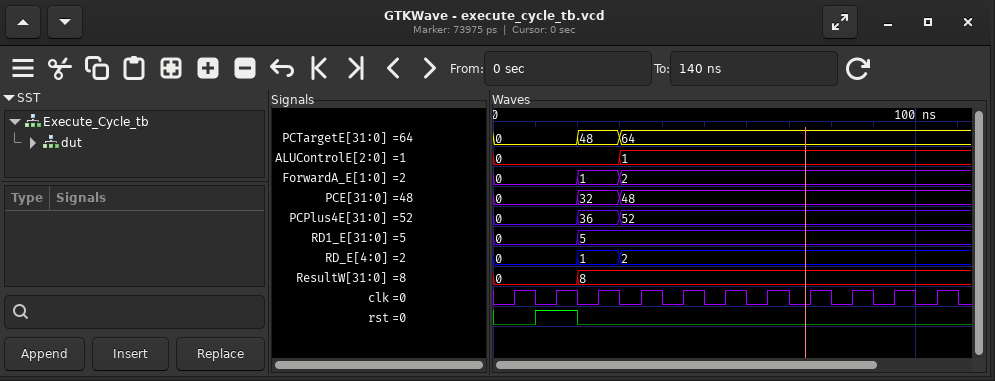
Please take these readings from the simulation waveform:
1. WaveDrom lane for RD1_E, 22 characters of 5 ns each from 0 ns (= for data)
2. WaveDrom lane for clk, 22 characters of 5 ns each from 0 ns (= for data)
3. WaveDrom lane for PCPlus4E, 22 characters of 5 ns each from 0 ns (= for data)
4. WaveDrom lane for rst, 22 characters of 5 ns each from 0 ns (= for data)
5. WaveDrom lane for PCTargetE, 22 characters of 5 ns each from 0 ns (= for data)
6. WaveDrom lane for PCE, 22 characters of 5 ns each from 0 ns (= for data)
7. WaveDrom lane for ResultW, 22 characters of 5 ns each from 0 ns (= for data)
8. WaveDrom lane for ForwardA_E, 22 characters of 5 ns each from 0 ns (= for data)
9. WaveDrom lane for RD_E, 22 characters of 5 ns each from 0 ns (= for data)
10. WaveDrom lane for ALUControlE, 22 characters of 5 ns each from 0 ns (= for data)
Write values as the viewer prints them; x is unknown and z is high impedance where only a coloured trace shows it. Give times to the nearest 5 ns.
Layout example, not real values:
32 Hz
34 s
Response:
{name: 'RD1_E', wave: '=...=.................', data: '0 5'}
{name: 'clk', wave: '0101010101010101010101'}
{name: 'PCPlus4E', wave: '=...=.=...............', data: '0 36 52'}
{name: 'rst', wave: '0.1.0.................'}
{name: 'PCTargetE', wave: '=...=.=...............', data: '0 48 64'}
{name: 'PCE', wave: '=...=.=...............', data: '0 32 48'}
{name: 'ResultW', wave: '=...=.................', data: '0 8'}
{name: 'ForwardA_E', wave: '=...=.=...............', data: '0 1 2'}
{name: 'RD_E', wave: '=...=.=...............', data: '0 1 2'}
{name: 'ALUControlE', wave: '=.....=...............', data: '0 1'}
